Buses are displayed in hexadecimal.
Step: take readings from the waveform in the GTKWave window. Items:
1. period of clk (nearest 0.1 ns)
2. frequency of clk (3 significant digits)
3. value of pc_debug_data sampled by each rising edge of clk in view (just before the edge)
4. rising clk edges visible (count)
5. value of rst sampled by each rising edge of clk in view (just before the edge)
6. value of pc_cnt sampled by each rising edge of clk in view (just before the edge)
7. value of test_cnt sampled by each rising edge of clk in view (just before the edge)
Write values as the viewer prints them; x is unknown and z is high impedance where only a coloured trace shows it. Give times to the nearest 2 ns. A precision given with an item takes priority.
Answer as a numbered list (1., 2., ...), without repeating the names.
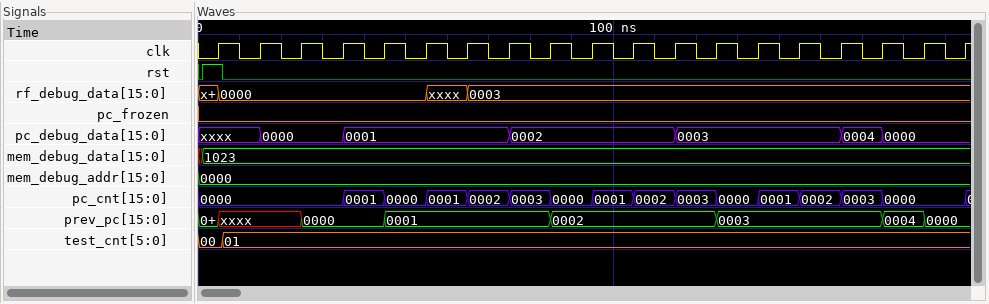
1. 10 ns
2. 100 MHz
3. xxxx, xxxx, 0000, 0000, 0001, 0001, 0001, 0001, 0002, 0002, 0002, 0002, 0003, 0003, 0003, 0003, 0004, 0000, 0000
4. 19
5. 1 0 0 0 0 0 0 0 0 0 0 0 0 0 0 0 0 0 0
6. 0000, 0000, 0000, 0000, 0001, 0000, 0001, 0002, 0003, 0000, 0001, 0002, 0003, 0000, 0001, 0002, 0003, 0000, 0000
7. 00, 01, 01, 01, 01, 01, 01, 01, 01, 01, 01, 01, 01, 01, 01, 01, 01, 01, 01
